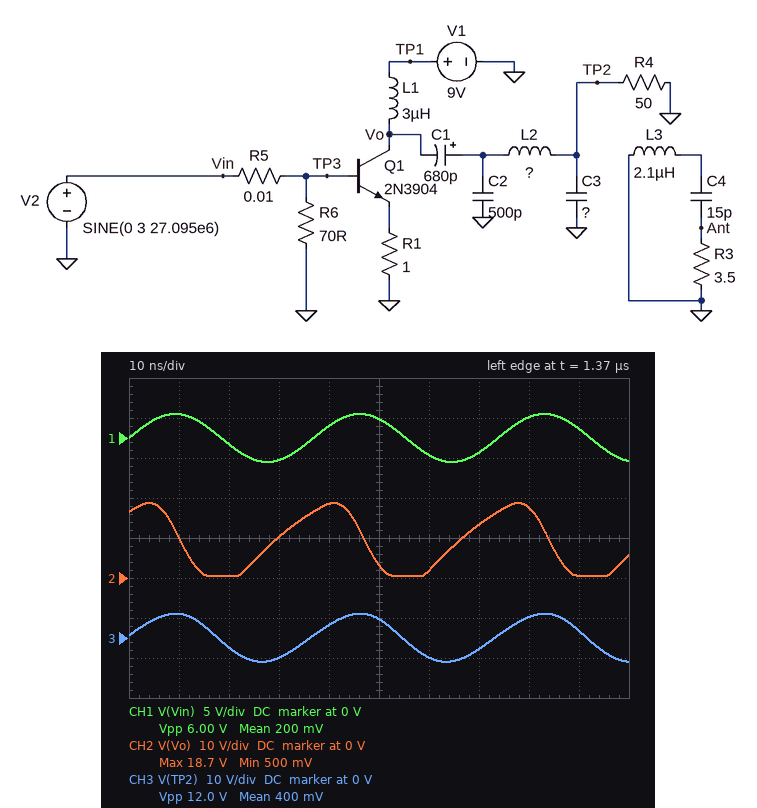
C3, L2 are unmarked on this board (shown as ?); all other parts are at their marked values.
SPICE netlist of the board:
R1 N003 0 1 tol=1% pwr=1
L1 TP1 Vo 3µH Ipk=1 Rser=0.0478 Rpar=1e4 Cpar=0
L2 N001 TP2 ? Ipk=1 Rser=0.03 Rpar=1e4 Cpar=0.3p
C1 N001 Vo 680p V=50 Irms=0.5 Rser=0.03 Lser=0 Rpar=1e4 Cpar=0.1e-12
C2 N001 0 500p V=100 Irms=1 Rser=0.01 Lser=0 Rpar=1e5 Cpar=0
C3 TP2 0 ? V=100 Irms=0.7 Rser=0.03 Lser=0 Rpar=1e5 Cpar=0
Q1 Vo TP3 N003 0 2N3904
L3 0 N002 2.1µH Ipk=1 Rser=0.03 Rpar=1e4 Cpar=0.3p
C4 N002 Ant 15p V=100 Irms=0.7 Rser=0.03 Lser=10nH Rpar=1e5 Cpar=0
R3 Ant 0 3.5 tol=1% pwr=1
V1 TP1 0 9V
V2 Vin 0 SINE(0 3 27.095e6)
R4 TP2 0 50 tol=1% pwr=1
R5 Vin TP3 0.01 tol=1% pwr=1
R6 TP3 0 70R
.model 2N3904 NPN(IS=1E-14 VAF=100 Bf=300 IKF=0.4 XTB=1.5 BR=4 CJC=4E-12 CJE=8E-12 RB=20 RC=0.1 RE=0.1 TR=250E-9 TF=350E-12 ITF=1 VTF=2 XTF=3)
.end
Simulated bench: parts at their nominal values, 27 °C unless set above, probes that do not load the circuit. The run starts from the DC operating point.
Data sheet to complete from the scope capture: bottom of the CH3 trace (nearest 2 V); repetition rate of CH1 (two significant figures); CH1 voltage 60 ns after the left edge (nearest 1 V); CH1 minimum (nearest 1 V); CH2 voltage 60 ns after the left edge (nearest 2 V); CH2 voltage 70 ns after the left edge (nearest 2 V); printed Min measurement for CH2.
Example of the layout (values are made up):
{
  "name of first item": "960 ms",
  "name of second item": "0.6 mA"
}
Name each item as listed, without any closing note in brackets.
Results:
{
  "bottom of the CH3 trace": "-6 V",
  "repetition rate of CH1": "27 MHz",
  "CH1 voltage 60 ns after the left edge": "-2 V",
  "CH1 minimum": "-3 V",
  "CH2 voltage 60 ns after the left edge": "2 V",
  "CH2 voltage 70 ns after the left edge": "14 V",
  "printed Min measurement for CH2": "500 mV"
}
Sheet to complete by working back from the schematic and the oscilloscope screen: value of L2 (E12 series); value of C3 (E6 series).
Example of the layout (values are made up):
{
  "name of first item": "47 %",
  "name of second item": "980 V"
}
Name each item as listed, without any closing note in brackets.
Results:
{
  "value of L2": "270 nH",
  "value of C3": "100 pF"
}
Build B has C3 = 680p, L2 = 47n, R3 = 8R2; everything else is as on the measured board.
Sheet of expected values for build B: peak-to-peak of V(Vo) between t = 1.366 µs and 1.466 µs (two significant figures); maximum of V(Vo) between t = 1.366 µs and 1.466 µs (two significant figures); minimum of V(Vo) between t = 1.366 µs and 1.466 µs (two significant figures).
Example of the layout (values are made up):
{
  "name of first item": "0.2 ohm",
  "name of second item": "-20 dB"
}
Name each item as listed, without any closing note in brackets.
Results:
{
  "peak-to-peak of V(Vo) between t = 1.366 µs and 1.466 µs": "13 V",
  "maximum of V(Vo) between t = 1.366 µs and 1.466 µs": "16 V",
  "minimum of V(Vo) between t = 1.366 µs and 1.466 µs": "2.7 V"
}
